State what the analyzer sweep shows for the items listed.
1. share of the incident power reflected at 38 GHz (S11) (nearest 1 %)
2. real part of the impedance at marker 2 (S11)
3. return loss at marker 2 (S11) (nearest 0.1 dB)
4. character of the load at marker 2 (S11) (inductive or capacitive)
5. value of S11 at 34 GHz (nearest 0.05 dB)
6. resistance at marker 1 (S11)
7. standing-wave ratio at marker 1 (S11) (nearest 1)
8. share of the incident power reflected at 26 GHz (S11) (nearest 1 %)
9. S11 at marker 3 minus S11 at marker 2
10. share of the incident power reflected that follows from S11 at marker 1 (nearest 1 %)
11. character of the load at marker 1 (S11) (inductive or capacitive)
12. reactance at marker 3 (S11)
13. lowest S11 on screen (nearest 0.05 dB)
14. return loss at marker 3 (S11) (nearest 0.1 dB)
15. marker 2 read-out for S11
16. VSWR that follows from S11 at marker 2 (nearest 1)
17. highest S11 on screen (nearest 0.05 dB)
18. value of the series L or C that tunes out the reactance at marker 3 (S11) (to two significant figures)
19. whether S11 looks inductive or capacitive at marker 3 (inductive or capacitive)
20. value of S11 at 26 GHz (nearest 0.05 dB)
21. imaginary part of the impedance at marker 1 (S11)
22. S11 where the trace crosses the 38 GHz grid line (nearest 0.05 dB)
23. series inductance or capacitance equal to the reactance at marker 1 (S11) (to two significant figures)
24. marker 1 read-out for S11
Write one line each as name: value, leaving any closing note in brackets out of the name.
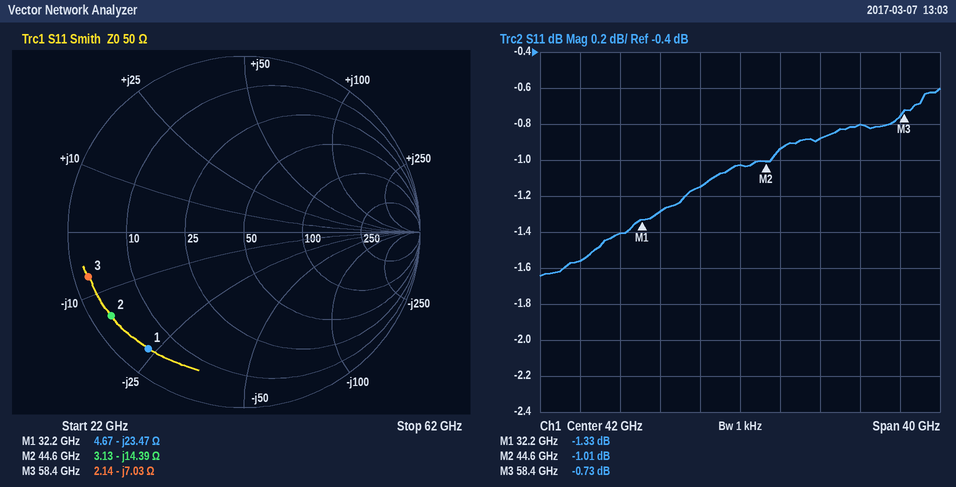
share of the incident power reflected at 38 GHz (S11): 77 %
real part of the impedance at marker 2: 3.13 Ω
return loss at marker 2 (S11): 1.0 dB
character of the load at marker 2 (S11): capacitive
value of S11 at 34 GHz: -1.30 dB
resistance at marker 1: 4.67 Ω
standing-wave ratio at marker 1 (S11): 13
share of the incident power reflected at 26 GHz (S11): 70 %
S11 at marker 3 minus S11 at marker 2: 0.28 dB
share of the incident power reflected that follows from S11 at marker 1: 74 %
character of the load at marker 1 (S11): capacitive
reactance at marker 3: -7.03 Ω
lowest S11 on screen: -1.65 dB
return loss at marker 3 (S11): 0.7 dB
marker 2 read-out for S11: -1.01 dB
VSWR that follows from S11 at marker 2: 17
highest S11 on screen: -0.60 dB
value of the series L or C that tunes out the reactance at marker 3 (S11): 19 pH
whether S11 looks inductive or capacitive at marker 3: capacitive
value of S11 at 26 GHz: -1.55 dB
imaginary part of the impedance at marker 1: -23.47 Ω
S11 where the trace crosses the 38 GHz grid line: -1.15 dB
series inductance or capacitance equal to the reactance at marker 1 (S11): 210 fF
marker 1 read-out for S11: -1.33 dB
